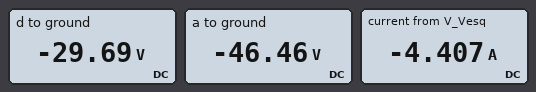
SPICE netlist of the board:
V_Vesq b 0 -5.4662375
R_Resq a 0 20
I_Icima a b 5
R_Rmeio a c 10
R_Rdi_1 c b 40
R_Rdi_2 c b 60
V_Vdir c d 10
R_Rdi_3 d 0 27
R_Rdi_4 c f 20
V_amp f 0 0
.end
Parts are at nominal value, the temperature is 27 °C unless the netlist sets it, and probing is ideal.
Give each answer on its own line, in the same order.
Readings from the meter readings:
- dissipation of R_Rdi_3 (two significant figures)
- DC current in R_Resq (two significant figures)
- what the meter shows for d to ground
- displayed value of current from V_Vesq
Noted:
33 W
2.3 A
-29.69 V
-4.407 A
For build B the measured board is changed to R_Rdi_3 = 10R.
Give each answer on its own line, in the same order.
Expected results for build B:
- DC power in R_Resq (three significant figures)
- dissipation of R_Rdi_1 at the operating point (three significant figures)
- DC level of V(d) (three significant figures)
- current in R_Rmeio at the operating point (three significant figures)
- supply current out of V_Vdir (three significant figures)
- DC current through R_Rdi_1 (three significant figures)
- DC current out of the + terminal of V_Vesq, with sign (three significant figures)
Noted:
83.7 W
875 mW
-21.4 V
2.95 A
2.14 A
148 mA
-4.75 A
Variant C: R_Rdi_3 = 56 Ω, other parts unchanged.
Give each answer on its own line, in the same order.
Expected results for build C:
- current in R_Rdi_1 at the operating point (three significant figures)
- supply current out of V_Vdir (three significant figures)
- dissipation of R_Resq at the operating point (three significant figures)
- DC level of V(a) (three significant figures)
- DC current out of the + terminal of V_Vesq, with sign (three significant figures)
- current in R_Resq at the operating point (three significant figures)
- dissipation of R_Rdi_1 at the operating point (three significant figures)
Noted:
455 mA
601 mA
121 W
-49.1 V
-4.24 A
2.46 A
8.29 W
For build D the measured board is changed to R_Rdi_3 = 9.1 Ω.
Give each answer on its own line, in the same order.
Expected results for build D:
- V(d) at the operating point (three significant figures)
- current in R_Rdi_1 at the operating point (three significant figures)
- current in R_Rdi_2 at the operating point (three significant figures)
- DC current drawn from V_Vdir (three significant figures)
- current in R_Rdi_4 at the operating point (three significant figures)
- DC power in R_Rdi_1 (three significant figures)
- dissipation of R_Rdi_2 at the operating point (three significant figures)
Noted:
-20.5 V
125 mA
83.6 mA
2.25 A
524 mA
629 mW
419 mW
